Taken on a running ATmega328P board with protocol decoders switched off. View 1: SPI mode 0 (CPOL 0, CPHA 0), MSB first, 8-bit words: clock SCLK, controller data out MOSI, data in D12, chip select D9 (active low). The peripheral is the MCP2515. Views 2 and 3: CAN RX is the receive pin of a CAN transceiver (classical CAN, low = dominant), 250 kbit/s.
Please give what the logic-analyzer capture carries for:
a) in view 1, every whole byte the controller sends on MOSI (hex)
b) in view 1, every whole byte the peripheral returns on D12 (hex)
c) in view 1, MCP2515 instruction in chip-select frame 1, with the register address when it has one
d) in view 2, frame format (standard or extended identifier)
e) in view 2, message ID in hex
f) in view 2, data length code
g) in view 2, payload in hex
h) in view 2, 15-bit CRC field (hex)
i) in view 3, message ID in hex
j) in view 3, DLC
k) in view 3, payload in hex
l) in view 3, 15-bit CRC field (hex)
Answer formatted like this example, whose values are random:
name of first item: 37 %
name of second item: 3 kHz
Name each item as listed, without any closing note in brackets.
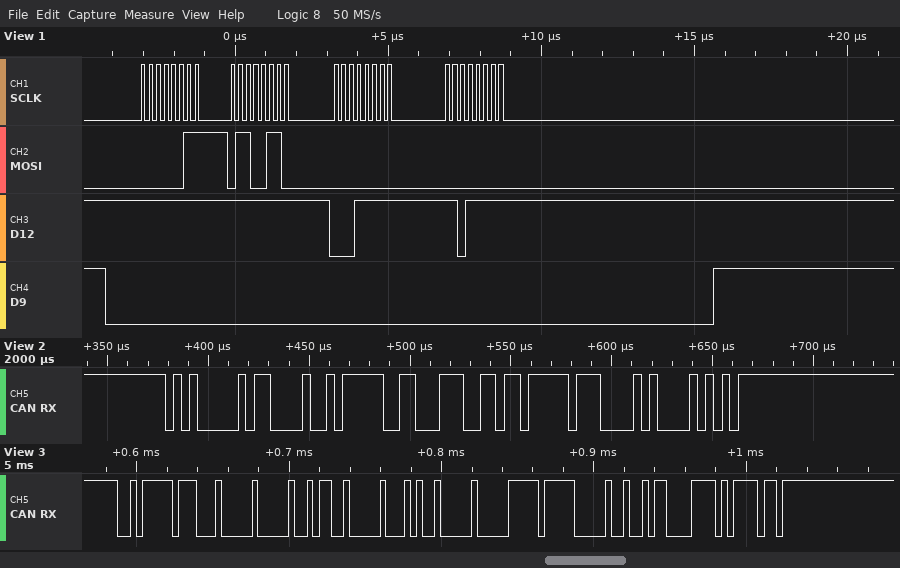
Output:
in view 1, every whole byte the controller sends on MOSI: 03 66 00 00
in view 1, every whole byte the peripheral returns on D12: FF FF 1F DF
in view 1, MCP2515 instruction in chip-select frame 1, with the register address when it has one: READ 0x66
in view 2, frame format: standard
in view 2, message ID in hex: 0x503
in view 2, data length code: 4
in view 2, payload in hex: BE C7 36 FF
in view 2, 15-bit CRC field: 0x050A
in view 3, message ID in hex: 0x2FF
in view 3, DLC: 8
in view 3, payload in hex: 00 59 00 A4 00 FF 81 2C
in view 3, 15-bit CRC field: 0x1EBD
